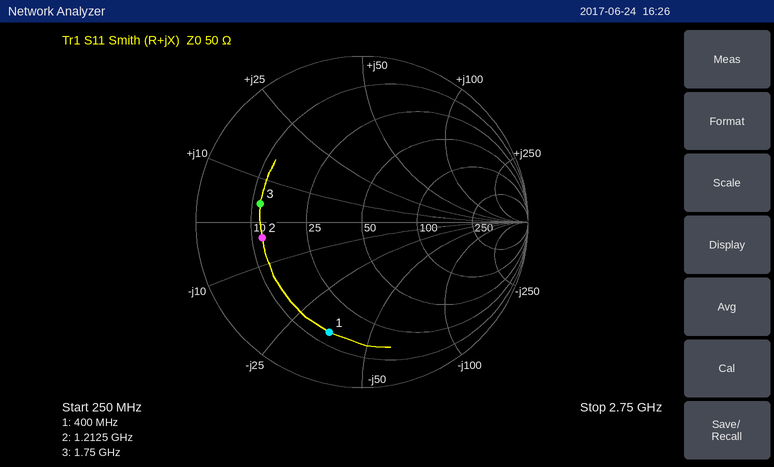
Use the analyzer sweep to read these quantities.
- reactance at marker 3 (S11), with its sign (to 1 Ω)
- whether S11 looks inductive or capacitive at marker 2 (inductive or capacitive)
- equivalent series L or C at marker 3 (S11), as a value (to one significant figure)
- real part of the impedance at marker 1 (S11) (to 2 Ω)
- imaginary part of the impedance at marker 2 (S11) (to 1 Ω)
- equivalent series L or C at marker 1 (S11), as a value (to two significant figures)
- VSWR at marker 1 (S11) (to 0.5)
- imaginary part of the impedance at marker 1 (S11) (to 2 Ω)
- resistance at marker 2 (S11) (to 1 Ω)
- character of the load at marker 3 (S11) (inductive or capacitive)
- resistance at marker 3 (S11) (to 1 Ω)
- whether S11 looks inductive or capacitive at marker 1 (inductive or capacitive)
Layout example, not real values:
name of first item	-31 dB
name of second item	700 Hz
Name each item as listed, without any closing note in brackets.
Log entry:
reactance at marker 3 (S11), with its sign	+4 Ω
whether S11 looks inductive or capacitive at marker 2	capacitive
equivalent series L or C at marker 3 (S11), as a value	400 pH
real part of the impedance at marker 1 (S11)	14 Ω
imaginary part of the impedance at marker 2 (S11)	-4 Ω
equivalent series L or C at marker 1 (S11), as a value	11 pF
VSWR at marker 1 (S11)	5.5
imaginary part of the impedance at marker 1 (S11)	-36 Ω
resistance at marker 2 (S11)	12 Ω
character of the load at marker 3 (S11)	inductive
resistance at marker 3 (S11)	12 Ω
whether S11 looks inductive or capacitive at marker 1	capacitive
